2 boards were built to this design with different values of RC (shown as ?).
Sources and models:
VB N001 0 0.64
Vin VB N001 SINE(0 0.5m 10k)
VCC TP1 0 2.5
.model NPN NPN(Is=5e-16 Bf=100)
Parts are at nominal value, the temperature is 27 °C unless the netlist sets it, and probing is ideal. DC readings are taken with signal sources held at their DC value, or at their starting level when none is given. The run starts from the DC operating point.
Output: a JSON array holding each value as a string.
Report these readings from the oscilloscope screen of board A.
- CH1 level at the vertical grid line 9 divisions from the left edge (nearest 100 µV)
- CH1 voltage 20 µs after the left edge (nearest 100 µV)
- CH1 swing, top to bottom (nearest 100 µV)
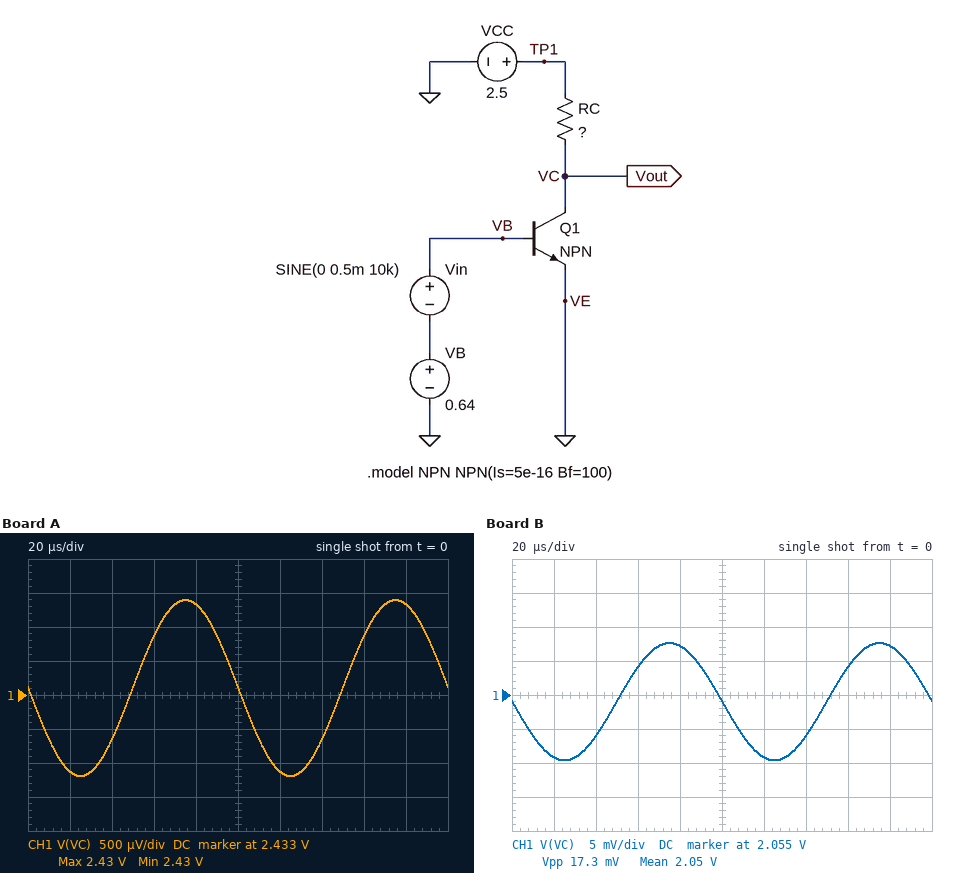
["2.4343 V", "2.4319 V", "2.6 mV"]
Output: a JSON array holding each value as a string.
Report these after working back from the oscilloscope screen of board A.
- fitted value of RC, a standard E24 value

["2.4 kΩ"]
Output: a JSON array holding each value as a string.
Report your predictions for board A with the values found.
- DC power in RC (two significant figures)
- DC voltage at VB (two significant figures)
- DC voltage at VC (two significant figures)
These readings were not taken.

["1.9 µW", "640 mV", "2.4 V"]
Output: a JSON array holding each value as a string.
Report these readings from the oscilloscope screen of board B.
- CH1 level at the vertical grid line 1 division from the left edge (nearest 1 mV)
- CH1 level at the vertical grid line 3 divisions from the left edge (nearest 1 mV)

["2.046 V", "2.059 V"]
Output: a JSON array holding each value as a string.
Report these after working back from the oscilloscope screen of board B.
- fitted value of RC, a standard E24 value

["16 kΩ"]
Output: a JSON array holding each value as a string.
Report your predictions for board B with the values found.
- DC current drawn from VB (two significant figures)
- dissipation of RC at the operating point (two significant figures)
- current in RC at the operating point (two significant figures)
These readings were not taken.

["280 nA", "12 µW", "28 µA"]
